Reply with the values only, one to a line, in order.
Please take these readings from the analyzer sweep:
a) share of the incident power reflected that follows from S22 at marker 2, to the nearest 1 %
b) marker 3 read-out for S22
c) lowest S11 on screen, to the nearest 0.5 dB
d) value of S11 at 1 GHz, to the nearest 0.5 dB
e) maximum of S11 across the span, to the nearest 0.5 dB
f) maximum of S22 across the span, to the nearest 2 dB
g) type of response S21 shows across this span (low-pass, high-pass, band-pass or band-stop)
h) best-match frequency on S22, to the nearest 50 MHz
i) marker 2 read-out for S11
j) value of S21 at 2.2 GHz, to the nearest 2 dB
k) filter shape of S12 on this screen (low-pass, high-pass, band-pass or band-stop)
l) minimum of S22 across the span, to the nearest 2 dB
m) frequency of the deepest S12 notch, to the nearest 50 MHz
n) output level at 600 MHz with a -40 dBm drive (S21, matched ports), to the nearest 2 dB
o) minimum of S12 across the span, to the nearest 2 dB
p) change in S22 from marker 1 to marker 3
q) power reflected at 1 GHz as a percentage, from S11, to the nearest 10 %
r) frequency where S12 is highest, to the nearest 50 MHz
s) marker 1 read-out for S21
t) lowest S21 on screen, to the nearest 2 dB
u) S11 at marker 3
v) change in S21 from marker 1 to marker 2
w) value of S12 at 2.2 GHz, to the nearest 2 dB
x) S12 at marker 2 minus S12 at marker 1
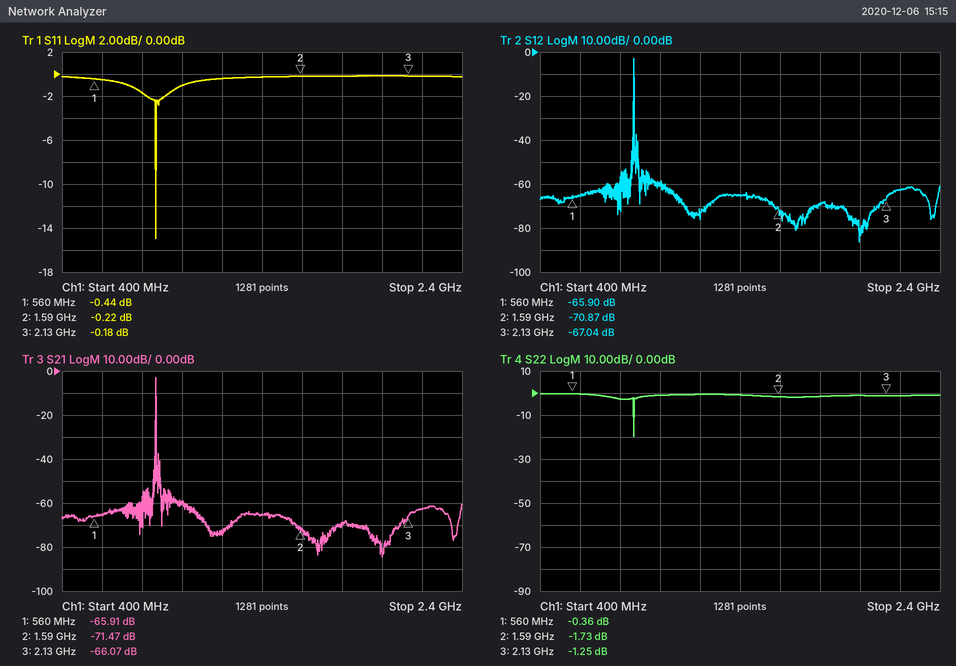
67 %
-1.25 dB
-15.0 dB
-1.0 dB
0.0 dB
0 dB
band-pass
850 MHz
-0.22 dB
-62 dB
band-pass
-20 dB
2.00 GHz
-106 dBm
-86 dB
-0.89 dB
80 %
850 MHz
-65.91 dB
-84 dB
-0.18 dB
-5.56 dB
-62 dB
-4.97 dB
